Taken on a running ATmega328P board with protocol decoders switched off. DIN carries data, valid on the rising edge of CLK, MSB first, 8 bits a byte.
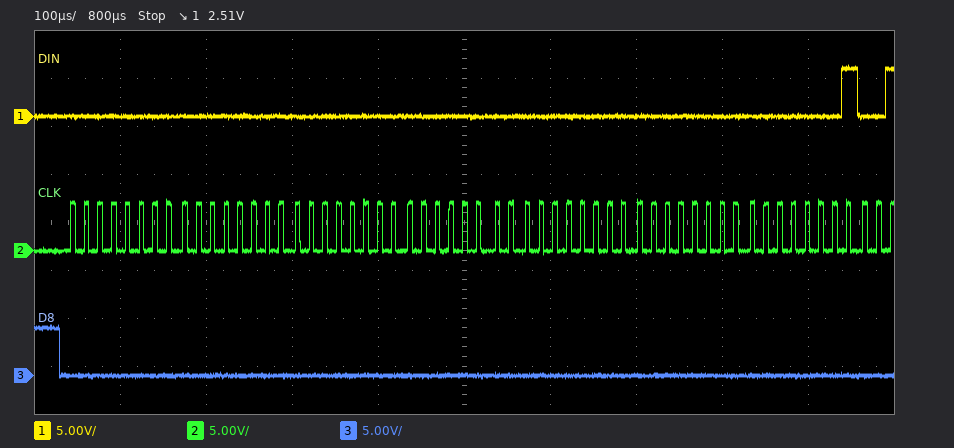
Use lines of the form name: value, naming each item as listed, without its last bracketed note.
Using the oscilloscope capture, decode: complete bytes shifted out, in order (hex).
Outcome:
complete bytes shifted out, in order: 0x00 0x00 0x00 0x00 0x00 0x00 0x01
